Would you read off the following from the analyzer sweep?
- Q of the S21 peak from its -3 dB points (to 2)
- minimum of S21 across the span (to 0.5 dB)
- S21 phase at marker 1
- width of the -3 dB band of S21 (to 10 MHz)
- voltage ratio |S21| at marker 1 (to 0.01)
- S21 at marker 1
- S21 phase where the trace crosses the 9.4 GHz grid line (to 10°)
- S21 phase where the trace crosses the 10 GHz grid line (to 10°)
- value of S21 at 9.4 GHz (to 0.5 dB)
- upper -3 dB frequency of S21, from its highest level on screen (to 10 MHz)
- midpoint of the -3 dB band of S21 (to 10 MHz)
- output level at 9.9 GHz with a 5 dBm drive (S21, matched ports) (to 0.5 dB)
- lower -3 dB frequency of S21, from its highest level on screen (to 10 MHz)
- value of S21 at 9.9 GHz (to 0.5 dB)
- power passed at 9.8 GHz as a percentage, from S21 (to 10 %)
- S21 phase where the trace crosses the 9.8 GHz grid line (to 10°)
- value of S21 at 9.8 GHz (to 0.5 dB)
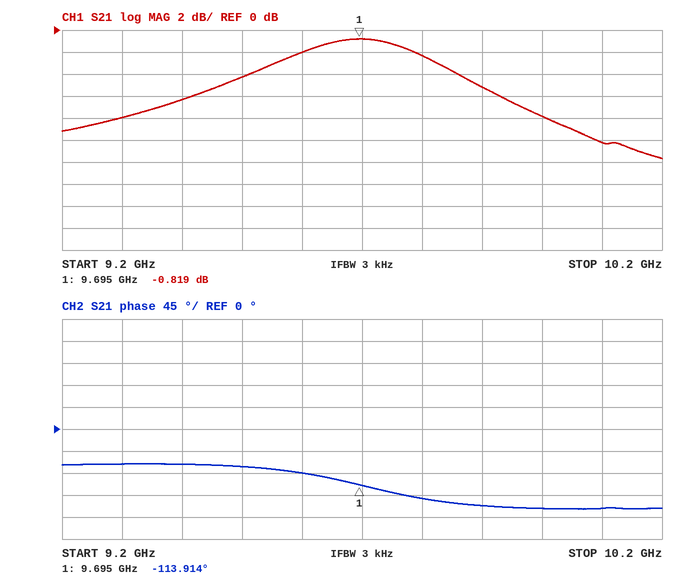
30
-11.5 dB
-113.914°
330 MHz
0.91
-0.819 dB
-70°
-160°
-6.5 dB
9.85 GHz
9.69 GHz
0.0 dBm
9.52 GHz
-5.0 dB
60 %
-140°
-2.5 dB
